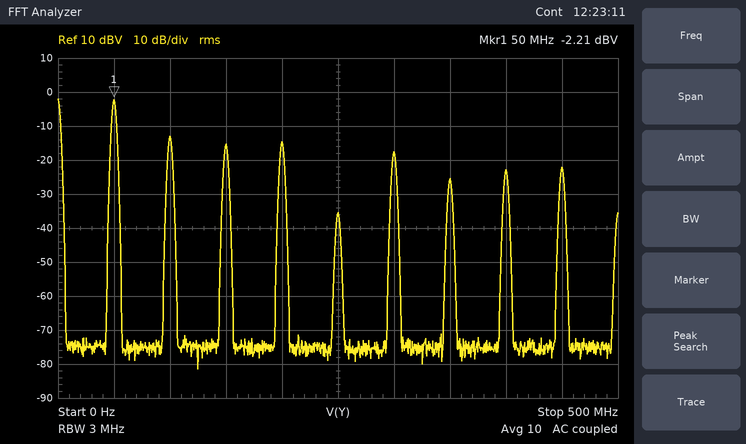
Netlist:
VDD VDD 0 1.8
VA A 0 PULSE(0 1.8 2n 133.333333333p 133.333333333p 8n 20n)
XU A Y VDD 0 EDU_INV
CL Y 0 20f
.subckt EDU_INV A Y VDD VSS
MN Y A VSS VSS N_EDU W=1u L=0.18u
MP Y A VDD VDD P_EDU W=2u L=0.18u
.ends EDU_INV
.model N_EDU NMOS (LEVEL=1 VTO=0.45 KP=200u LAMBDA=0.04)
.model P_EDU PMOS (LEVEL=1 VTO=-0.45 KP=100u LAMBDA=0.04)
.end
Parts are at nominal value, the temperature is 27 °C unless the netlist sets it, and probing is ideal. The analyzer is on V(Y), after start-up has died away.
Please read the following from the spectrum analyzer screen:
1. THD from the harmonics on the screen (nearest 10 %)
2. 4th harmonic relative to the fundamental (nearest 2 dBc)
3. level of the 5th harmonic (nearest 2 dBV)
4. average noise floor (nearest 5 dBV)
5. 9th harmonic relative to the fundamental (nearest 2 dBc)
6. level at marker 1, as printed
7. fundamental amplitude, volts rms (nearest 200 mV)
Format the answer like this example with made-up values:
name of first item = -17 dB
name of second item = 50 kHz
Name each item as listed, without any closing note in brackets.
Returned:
THD from the harmonics on the screen = 50 %
4th harmonic relative to the fundamental = -12 dBc
level of the 5th harmonic = -36 dBV
average noise floor = -75 dBV
9th harmonic relative to the fundamental = -20 dBc
level at marker 1, as printed = -2.21 dBV
fundamental amplitude, volts rms = 800 mV
